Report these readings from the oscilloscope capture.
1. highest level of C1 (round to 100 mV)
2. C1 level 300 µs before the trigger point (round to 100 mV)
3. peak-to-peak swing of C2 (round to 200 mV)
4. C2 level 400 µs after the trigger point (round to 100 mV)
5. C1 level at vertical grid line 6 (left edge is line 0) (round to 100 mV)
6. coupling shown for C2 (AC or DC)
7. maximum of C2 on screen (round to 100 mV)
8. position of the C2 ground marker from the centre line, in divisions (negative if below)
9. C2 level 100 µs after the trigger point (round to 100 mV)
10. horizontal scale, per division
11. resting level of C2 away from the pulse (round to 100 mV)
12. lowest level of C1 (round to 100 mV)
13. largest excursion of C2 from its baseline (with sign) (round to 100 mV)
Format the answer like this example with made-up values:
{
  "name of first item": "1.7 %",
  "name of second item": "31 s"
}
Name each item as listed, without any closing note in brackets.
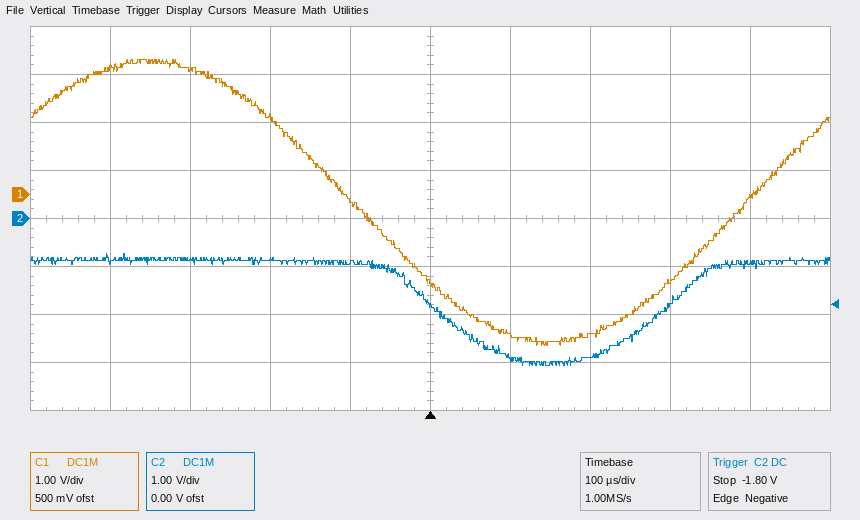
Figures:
{
  "highest level of C1": "2.8 V",
  "C1 level 300 µs before the trigger point": "2.6 V",
  "peak-to-peak swing of C2": "2.4 V",
  "C2 level 400 µs after the trigger point": "-900 mV",
  "C1 level at vertical grid line 6 (left edge is line 0)": "-2.9 V",
  "coupling shown for C2": "DC",
  "maximum of C2 on screen": "-700 mV",
  "position of the C2 ground marker from the centre line, in divisions": "0.0 div",
  "C2 level 100 µs after the trigger point": "-2.9 V",
  "horizontal scale, per division": "100 µs",
  "resting level of C2 away from the pulse": "-900 mV",
  "lowest level of C1": "-3.1 V",
  "largest excursion of C2 from its baseline (with sign)": "-2.2 V"
}
